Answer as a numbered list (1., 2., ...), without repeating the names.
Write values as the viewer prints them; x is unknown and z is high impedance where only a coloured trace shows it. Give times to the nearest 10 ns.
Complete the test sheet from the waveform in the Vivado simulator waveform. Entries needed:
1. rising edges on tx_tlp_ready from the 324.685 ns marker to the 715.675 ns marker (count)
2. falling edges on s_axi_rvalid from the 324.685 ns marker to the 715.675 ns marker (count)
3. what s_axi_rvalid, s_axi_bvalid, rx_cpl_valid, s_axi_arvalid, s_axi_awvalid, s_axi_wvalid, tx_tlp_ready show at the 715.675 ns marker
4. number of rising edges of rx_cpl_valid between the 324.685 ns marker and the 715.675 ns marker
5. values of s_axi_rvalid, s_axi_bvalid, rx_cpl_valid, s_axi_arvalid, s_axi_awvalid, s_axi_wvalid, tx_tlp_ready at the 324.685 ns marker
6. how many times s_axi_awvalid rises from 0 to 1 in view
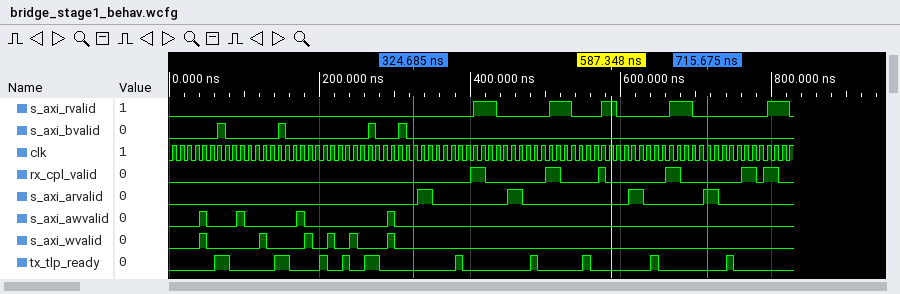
1. 4
2. 4
3. s_axi_rvalid=0, s_axi_bvalid=0, rx_cpl_valid=0, s_axi_arvalid=1, s_axi_awvalid=0, s_axi_wvalid=0, tx_tlp_ready=0
4. 4
5. s_axi_rvalid=0, s_axi_bvalid=0, rx_cpl_valid=0, s_axi_arvalid=0, s_axi_awvalid=0, s_axi_wvalid=0, tx_tlp_ready=0
6. 4
